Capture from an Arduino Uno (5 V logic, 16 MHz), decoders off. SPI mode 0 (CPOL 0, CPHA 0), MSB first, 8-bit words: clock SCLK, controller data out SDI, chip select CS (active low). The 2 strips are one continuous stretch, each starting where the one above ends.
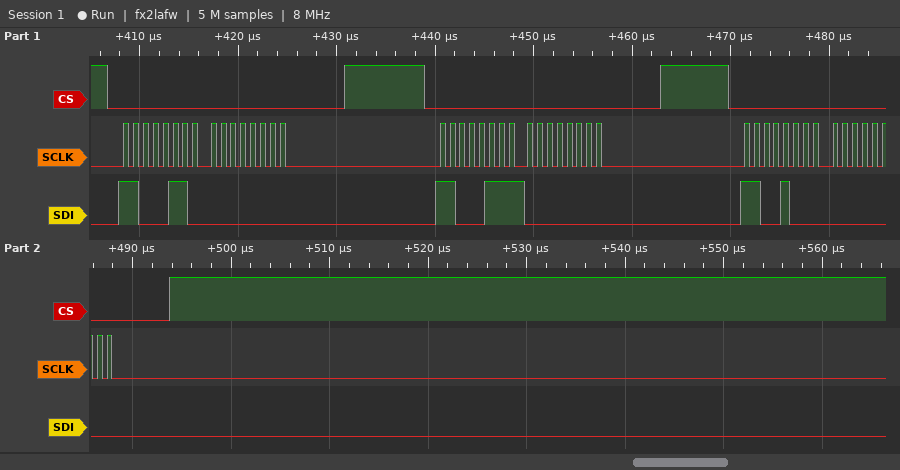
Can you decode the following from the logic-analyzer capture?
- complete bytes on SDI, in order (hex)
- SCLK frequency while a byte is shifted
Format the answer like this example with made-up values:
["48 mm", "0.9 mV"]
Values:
["C6 00 C7 00 C8 00", "1 MHz"]
